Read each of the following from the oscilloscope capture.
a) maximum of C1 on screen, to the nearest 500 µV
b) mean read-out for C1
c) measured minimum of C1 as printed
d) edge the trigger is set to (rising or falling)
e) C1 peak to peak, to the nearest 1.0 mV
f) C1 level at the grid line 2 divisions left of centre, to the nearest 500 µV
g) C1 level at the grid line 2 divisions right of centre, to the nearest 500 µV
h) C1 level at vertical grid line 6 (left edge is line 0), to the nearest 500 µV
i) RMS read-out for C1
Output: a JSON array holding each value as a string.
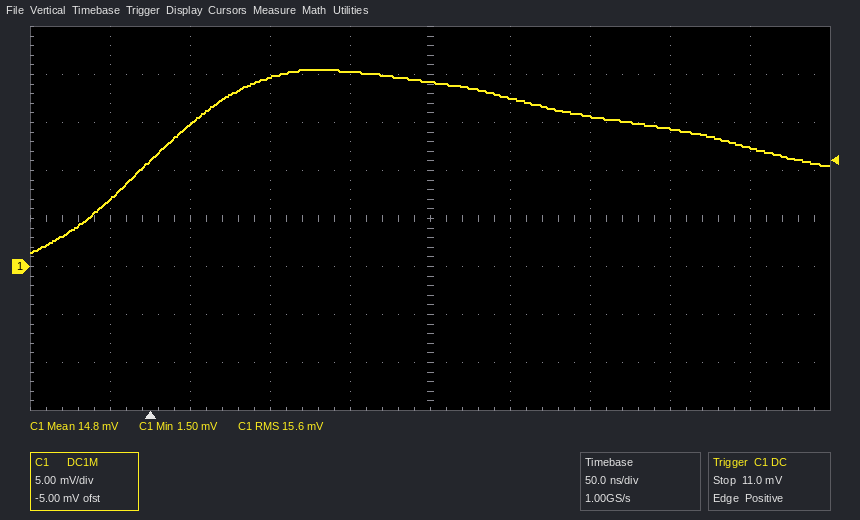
["20.5 mV", "14.8 mV", "1.50 mV", "rising", "19.0 mV", "19.5 mV", "15.5 mV", "17.5 mV", "15.6 mV"]
